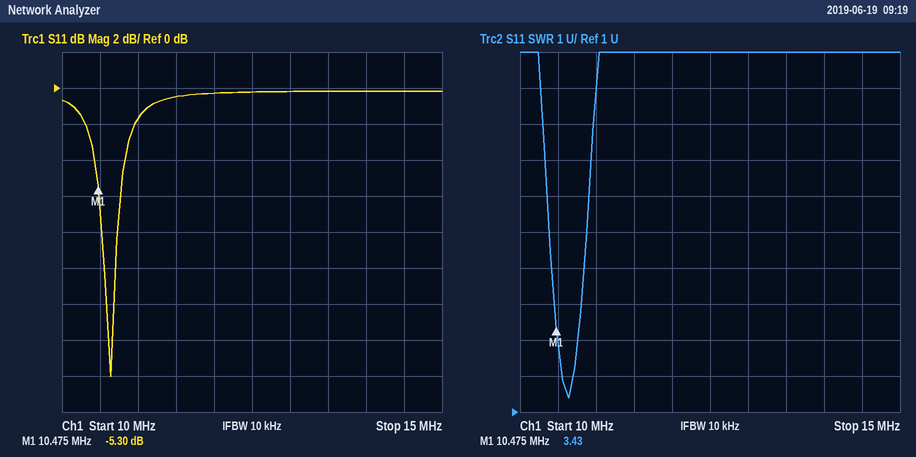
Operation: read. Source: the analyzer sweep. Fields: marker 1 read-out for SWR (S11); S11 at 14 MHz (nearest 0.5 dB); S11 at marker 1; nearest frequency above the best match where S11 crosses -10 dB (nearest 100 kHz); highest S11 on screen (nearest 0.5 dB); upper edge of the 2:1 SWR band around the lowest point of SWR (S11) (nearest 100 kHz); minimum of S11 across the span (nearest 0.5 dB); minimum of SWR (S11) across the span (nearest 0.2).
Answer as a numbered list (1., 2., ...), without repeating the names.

1. 3.43
2. 0.0 dB
3. -5.30 dB
4. 10.7 MHz
5. 0.0 dB
6. 10.7 MHz
7. -16.0 dB
8. 1.4
